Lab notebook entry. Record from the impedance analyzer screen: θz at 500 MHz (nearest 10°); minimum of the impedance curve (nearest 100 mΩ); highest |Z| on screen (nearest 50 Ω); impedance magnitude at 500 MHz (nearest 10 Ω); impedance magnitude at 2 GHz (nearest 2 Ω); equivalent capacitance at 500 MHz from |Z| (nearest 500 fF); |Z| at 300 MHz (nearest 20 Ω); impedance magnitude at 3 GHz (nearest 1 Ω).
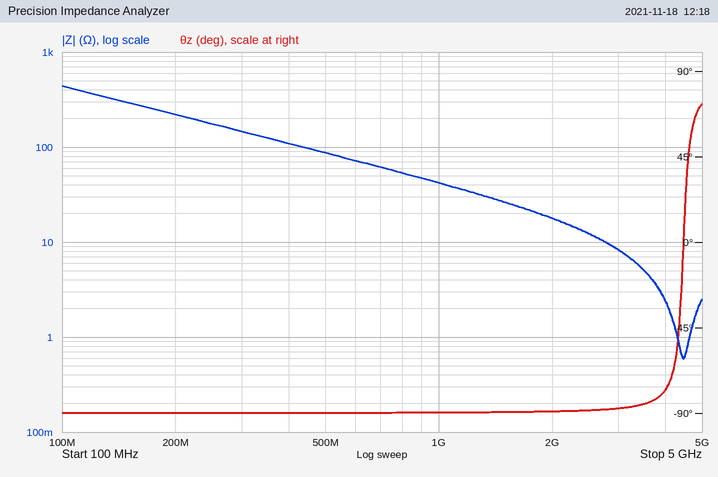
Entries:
-90°
600 mΩ
450 Ω
90 Ω
18 Ω
3.5 pF
140 Ω
8 Ω
